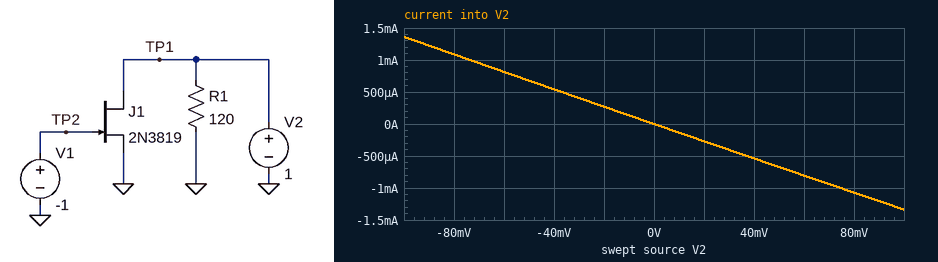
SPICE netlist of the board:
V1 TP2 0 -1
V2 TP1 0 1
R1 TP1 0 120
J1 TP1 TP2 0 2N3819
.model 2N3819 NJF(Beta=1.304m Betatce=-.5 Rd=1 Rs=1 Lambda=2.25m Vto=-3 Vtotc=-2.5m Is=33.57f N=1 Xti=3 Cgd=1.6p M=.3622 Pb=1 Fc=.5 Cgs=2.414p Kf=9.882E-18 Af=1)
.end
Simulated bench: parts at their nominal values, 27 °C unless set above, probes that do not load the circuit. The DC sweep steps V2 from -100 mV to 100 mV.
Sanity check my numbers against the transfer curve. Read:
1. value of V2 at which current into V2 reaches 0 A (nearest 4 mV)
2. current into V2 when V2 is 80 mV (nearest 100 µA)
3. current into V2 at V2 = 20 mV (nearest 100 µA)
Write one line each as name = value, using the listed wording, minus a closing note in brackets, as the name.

value of V2 at which current into V2 reaches 0 A = 0 V
current into V2 when V2 is 80 mV = -1.1 mA
current into V2 at V2 = 20 mV = -300 µA
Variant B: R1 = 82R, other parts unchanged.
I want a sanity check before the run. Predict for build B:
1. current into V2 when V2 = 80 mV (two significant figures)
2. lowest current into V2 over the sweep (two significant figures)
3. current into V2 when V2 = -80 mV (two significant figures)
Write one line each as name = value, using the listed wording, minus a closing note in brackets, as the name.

current into V2 when V2 = 80 mV = -1.4 mA
lowest current into V2 over the sweep = -1.7 mA
current into V2 when V2 = -80 mV = 1.4 mA
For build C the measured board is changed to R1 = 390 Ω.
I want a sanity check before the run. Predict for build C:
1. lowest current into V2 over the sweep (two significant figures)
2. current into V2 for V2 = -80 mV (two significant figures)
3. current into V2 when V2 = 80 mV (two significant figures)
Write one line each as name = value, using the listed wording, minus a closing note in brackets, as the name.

lowest current into V2 over the sweep = -760 µA
current into V2 for V2 = -80 mV = 630 µA
current into V2 when V2 = 80 mV = -610 µA
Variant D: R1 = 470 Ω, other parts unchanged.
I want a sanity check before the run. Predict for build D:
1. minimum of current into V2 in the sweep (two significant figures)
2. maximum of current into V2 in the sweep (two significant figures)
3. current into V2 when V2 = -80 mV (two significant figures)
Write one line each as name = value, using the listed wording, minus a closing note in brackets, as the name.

minimum of current into V2 in the sweep = -720 µA
maximum of current into V2 in the sweep = 740 µA
current into V2 when V2 = -80 mV = 590 µA
